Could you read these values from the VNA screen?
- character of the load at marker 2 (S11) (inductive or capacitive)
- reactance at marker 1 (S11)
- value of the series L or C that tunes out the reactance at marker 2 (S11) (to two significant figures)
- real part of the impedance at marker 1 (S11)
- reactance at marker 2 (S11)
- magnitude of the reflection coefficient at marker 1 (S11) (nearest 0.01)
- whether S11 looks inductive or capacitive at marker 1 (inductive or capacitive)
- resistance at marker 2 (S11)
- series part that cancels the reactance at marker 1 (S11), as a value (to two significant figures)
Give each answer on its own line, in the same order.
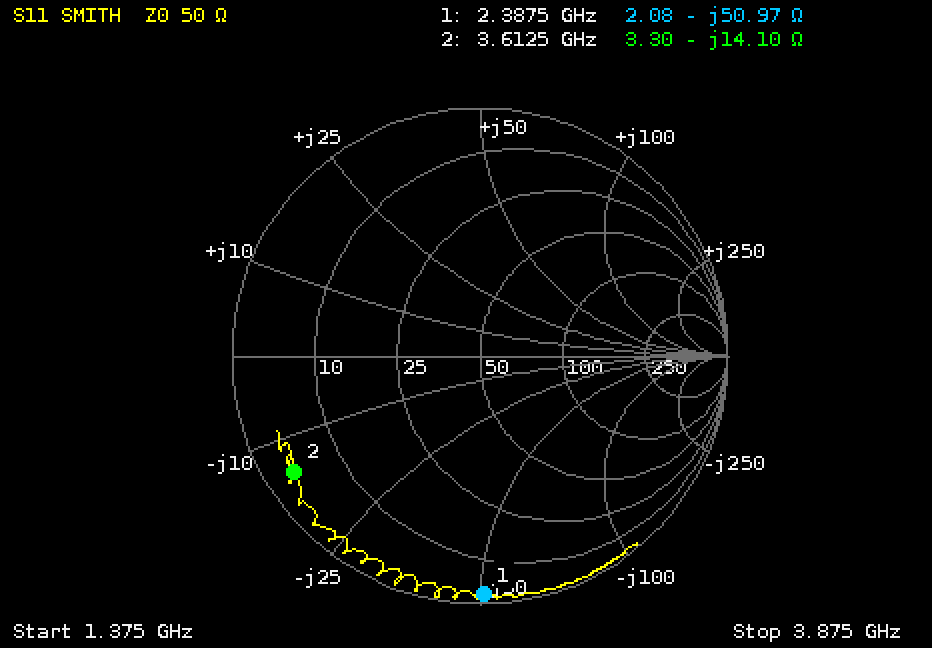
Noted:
capacitive
-50.97 Ω
620 pH
2.08 Ω
-14.10 Ω
0.96
capacitive
3.30 Ω
3.4 nH
